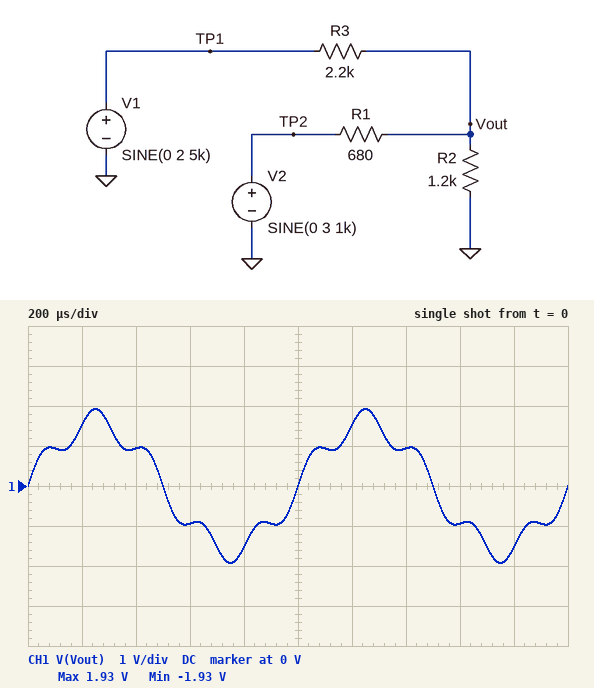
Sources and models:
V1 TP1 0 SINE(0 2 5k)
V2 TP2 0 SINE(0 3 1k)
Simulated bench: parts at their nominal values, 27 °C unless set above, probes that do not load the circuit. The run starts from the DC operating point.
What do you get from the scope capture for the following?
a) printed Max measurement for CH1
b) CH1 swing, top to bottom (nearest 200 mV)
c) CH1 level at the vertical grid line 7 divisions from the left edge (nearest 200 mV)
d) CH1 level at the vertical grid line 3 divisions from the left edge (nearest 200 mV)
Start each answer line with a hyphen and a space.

- 1.93 V
- 3.8 V
- 1.0 V
- -1.0 V
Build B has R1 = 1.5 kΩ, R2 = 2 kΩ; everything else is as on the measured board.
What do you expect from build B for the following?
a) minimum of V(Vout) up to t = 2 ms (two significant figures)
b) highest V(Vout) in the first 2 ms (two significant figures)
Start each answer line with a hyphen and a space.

- -1.8 V
- 1.8 V
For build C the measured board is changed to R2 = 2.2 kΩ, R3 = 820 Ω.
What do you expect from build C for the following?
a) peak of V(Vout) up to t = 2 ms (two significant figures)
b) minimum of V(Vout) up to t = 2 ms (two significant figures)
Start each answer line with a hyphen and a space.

- 2.2 V
- -2.2 V
